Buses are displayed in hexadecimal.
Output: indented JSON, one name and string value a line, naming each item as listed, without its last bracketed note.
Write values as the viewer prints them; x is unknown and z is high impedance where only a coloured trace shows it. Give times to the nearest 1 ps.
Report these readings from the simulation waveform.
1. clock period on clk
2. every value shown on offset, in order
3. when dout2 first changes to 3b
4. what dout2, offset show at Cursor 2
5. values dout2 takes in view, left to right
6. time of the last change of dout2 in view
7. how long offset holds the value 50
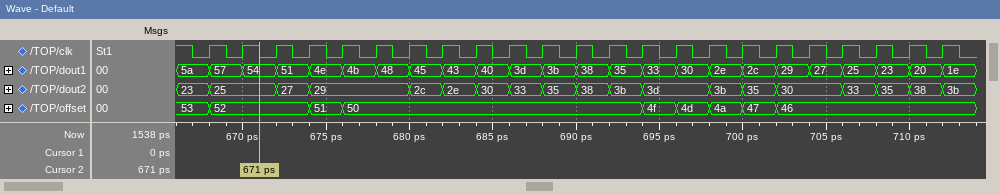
{
  "clock period on clk": "2 ps",
  "every value shown on offset, in order": "53, 52, 51, 50, 4f, 4d, 4a, 47, 46",
  "when dout2 first changes to 3b": "692 ps",
  "what dout2, offset show at Cursor 2": "dout2=25, offset=52",
  "values dout2 takes in view, left to right": "23, 25, 27, 29, 2c, 2e, 30, 33, 35, 38, 3b, 3d, 3b, 35, 30, 33, 35, 38, 3b",
  "time of the last change of dout2 in view": "712 ps",
  "how long offset holds the value 50": "18 ps"
}
